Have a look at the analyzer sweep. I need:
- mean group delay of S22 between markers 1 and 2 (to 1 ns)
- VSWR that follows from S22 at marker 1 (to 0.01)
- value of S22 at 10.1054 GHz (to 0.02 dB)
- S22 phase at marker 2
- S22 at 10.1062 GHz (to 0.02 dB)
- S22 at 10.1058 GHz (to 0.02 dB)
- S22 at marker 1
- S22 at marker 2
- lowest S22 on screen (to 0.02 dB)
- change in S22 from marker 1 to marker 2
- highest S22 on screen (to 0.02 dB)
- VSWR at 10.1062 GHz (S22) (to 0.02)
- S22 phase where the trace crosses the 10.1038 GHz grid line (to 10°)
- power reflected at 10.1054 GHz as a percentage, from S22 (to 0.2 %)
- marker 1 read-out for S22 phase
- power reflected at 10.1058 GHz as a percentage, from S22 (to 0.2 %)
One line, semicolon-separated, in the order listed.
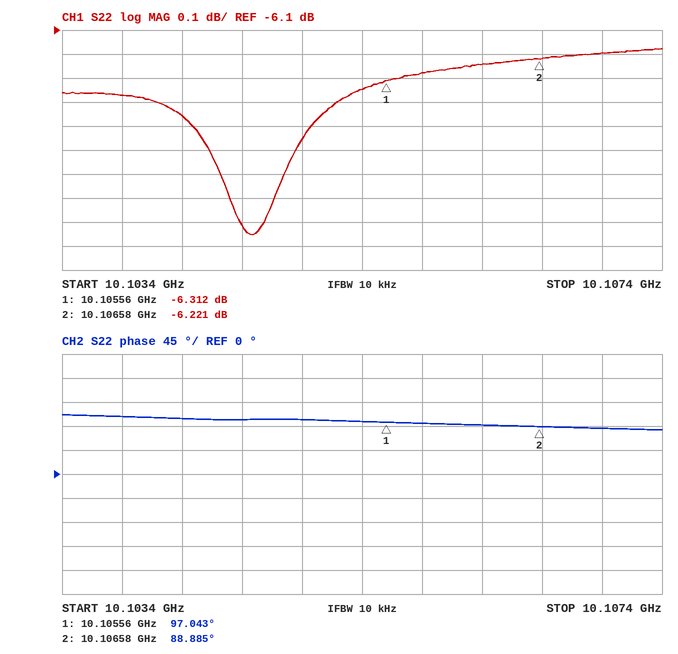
22 ns; 2.87; -6.34 dB; 88.885°; -6.24 dB; -6.28 dB; -6.312 dB; -6.221 dB; -6.96 dB; 0.091 dB; -6.18 dB; 2.90; 110°; 23.2 %; 97.043°; 23.6 %
